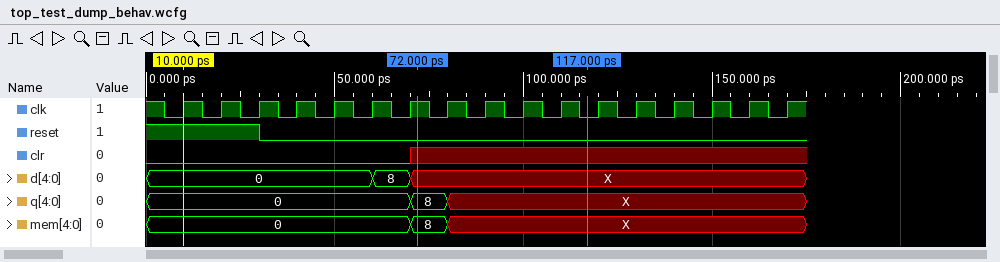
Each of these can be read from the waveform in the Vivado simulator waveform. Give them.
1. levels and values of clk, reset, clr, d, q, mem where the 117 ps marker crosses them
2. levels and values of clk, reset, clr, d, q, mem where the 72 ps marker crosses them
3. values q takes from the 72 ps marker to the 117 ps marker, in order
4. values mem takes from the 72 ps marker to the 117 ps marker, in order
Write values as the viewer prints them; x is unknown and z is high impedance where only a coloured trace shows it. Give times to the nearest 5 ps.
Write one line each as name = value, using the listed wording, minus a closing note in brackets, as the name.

levels and values of clk, reset, clr, d, q, mem where the 117 ps marker crosses them = clk=0, reset=0, clr=x, d=X, q=X, mem=X
levels and values of clk, reset, clr, d, q, mem where the 72 ps marker crosses them = clk=1, reset=0, clr=x, d=X, q=8, mem=8
values q takes from the 72 ps marker to the 117 ps marker, in order = 8, X
values mem takes from the 72 ps marker to the 117 ps marker, in order = 8, X
